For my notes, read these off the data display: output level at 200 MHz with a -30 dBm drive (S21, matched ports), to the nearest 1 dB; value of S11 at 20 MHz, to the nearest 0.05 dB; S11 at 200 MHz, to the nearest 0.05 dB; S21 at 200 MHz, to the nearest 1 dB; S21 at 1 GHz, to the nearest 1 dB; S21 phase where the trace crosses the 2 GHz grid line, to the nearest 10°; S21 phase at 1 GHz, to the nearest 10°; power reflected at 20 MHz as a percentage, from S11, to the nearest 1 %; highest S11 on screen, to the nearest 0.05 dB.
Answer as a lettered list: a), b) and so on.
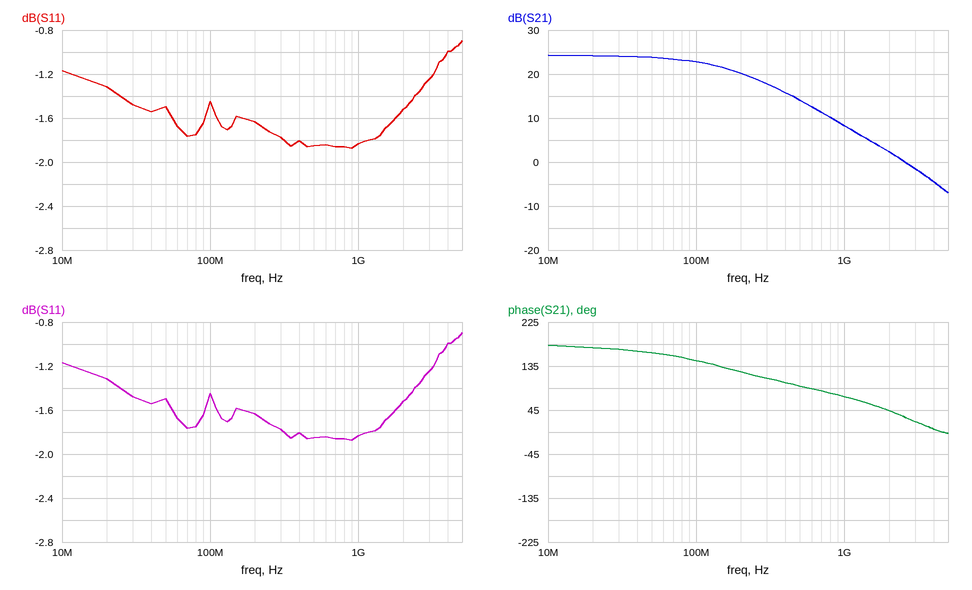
a) -10 dBm
b) -1.30 dB
c) -1.65 dB
d) 20 dB
e) 8 dB
f) 40°
g) 70°
h) 74 %
i) -0.90 dB
